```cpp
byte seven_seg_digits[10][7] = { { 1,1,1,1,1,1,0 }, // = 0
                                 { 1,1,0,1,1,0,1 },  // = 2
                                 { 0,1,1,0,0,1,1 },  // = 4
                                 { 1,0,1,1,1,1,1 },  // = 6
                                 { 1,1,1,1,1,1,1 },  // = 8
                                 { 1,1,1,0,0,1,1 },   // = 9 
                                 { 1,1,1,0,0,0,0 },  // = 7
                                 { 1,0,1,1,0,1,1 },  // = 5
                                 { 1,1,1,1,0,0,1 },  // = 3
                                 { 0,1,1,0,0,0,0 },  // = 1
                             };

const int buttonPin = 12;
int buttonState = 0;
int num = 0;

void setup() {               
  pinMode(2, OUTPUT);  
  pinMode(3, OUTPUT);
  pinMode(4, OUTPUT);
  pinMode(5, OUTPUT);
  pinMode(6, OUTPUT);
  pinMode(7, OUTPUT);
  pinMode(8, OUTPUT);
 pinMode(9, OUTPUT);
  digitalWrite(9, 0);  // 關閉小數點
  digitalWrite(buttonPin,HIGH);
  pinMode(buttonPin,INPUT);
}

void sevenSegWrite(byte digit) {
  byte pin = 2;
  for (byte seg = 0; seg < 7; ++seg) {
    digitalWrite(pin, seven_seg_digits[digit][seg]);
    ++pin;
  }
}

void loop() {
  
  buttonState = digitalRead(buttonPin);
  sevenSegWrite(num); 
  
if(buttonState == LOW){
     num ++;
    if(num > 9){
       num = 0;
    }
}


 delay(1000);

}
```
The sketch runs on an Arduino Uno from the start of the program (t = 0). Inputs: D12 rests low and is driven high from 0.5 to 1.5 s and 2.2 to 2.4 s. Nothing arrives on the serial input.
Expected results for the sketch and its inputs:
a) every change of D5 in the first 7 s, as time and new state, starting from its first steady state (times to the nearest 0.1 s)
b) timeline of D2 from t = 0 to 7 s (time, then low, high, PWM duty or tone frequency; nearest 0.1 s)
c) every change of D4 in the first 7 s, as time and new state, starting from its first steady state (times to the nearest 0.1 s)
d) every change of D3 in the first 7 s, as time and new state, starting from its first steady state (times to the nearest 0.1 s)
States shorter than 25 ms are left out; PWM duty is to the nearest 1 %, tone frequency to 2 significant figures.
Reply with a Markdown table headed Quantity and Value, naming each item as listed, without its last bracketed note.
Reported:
| Quantity | Value |
|---|---|
| every change of D5 in the first 7 s, as time and new state, starting from its first steady state | 0 s high; 3 s low; 4 s high; 6 s low |
| timeline of D2 from t = 0 to 7 s | 0 s high; 3 s low; 4 s high |
| every change of D4 in the first 7 s, as time and new state, starting from its first steady state | 0 s high; 1 s low; 3 s high |
| every change of D3 in the first 7 s, as time and new state, starting from its first steady state | 0 s high; 4 s low; 5 s high |
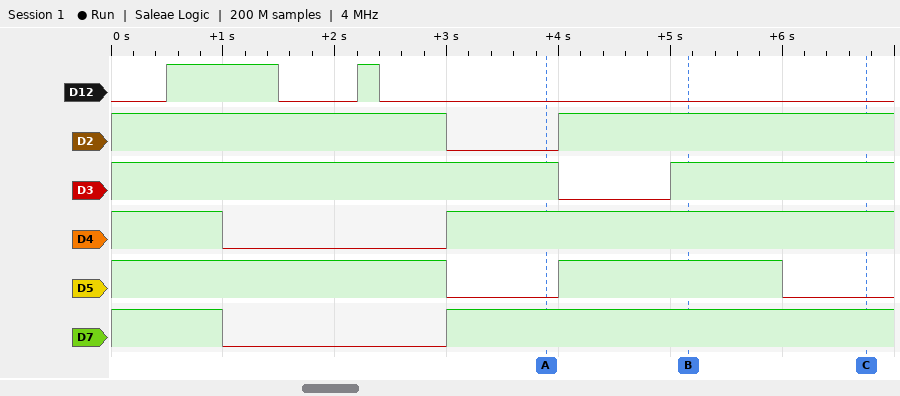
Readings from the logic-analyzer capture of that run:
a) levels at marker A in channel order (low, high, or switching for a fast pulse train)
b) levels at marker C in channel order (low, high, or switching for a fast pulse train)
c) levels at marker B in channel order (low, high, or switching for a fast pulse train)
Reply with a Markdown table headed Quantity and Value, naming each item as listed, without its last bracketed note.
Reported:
| Quantity | Value |
|---|---|
| levels at marker A in channel order | D12 low, D2 low, D3 high, D4 high, D5 low, D7 high |
| levels at marker C in channel order | D12 low, D2 high, D3 high, D4 high, D5 low, D7 high |
| levels at marker B in channel order | D12 low, D2 high, D3 high, D4 high, D5 high, D7 high |
